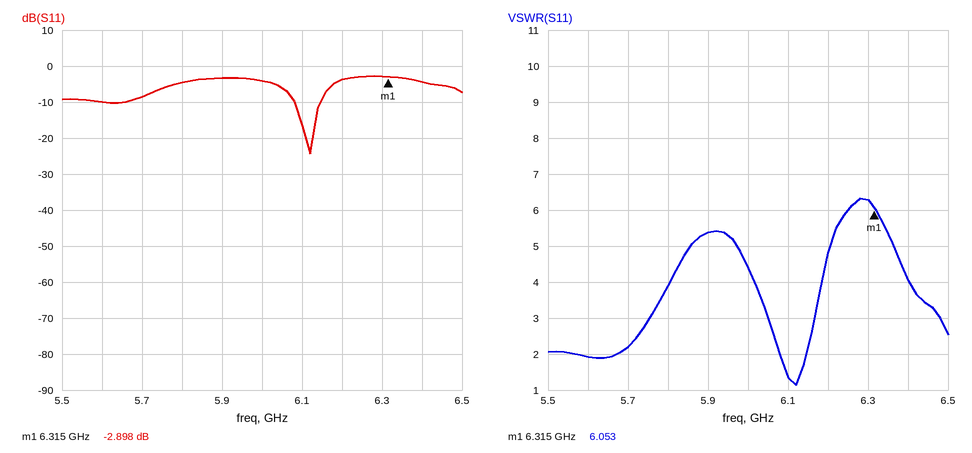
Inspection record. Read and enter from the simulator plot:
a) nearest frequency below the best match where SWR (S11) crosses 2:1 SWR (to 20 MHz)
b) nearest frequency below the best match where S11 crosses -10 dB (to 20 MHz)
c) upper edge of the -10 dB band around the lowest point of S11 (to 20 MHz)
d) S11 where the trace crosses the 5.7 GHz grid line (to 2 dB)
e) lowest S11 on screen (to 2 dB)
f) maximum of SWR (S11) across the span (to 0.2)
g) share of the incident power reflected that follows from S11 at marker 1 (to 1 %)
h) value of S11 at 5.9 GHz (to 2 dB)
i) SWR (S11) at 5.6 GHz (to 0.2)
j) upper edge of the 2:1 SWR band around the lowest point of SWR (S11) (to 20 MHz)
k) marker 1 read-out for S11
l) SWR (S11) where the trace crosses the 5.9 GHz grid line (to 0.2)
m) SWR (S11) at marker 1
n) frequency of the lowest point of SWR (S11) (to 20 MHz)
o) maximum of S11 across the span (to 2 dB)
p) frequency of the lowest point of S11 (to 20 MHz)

6.08 GHz
6.08 GHz
6.14 GHz
-8 dB
-24 dB
6.4
51 %
-4 dB
2.0
6.14 GHz
-2.898 dB
5.4
6.053
6.12 GHz
-2 dB
6.12 GHz
